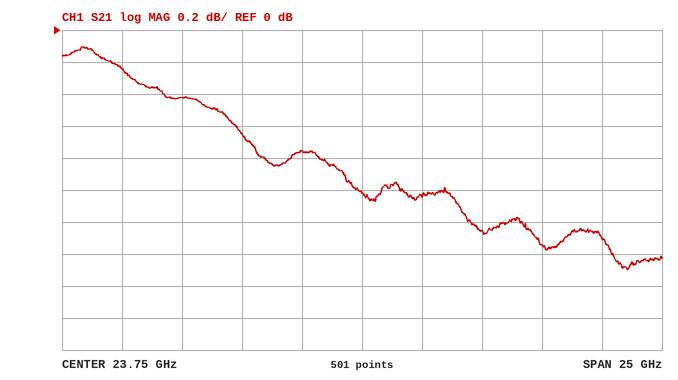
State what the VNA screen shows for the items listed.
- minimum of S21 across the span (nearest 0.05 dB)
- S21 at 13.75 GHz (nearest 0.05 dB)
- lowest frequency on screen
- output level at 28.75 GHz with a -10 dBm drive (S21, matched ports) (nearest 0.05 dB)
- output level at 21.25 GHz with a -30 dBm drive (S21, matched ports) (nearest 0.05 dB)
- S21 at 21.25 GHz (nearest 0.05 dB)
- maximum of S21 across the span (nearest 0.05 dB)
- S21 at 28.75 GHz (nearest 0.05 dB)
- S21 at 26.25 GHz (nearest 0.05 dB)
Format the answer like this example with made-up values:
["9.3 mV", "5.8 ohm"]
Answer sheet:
["-1.50 dB", "-0.25 dB", "11.25 GHz", "-11.25 dBm", "-30.75 dBm", "-0.75 dB", "-0.10 dB", "-1.25 dB", "-1.05 dB"]
